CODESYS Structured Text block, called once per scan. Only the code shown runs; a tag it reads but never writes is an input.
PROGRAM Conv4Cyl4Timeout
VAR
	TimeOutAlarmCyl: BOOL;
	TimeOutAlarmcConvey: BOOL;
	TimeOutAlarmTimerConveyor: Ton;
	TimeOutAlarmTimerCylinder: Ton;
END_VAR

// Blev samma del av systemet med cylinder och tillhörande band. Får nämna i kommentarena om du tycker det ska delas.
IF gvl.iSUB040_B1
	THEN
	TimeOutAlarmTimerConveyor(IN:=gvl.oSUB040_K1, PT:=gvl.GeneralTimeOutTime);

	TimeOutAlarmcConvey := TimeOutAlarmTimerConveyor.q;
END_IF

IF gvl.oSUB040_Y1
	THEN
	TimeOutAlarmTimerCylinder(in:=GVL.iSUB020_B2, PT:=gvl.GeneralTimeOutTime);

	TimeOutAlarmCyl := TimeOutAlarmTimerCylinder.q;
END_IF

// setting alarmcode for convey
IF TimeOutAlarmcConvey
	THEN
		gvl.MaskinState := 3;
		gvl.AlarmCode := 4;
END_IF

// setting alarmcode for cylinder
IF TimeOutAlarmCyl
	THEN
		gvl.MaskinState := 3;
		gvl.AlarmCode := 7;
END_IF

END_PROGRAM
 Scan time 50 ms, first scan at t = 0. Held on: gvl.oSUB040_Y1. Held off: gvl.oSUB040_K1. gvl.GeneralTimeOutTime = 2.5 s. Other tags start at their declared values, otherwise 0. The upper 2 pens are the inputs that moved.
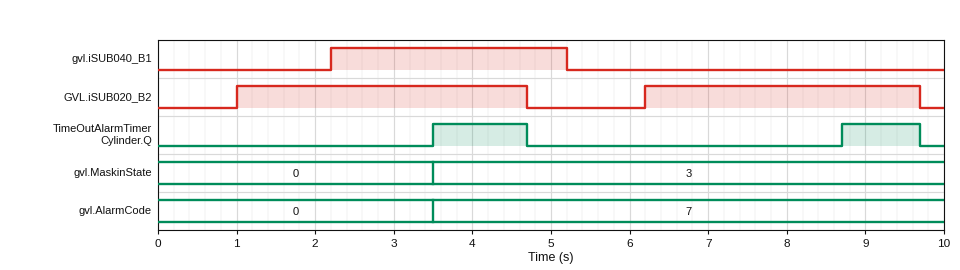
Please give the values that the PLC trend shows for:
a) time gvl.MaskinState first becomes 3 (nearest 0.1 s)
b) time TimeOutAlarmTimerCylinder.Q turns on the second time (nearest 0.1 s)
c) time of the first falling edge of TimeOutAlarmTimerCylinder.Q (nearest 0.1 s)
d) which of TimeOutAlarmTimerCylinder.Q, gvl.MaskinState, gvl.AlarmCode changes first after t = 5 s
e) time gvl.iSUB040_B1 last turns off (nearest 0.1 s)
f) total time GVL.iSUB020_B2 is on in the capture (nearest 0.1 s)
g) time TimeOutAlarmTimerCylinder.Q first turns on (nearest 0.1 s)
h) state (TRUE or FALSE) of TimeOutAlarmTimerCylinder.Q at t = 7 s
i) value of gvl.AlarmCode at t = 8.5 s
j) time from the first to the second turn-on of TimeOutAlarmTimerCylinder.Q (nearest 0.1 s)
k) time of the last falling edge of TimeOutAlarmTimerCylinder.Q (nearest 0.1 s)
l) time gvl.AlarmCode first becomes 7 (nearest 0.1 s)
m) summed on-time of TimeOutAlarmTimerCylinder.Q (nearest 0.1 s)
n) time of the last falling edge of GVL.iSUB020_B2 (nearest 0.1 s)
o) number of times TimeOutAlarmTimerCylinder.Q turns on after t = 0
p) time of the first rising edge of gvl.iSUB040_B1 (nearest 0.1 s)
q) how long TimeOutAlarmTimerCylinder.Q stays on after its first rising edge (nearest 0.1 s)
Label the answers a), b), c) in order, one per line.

a) 3.5 s
b) 8.7 s
c) 4.7 s
d) TimeOutAlarmTimerCylinder.Q
e) 5.2 s
f) 7.2 s
g) 3.5 s
h) FALSE
i) 7
j) 5.2 s
k) 9.7 s
l) 3.5 s
m) 2.2 s
n) 9.7 s
o) 2
p) 2.2 s
q) 1.2 s
